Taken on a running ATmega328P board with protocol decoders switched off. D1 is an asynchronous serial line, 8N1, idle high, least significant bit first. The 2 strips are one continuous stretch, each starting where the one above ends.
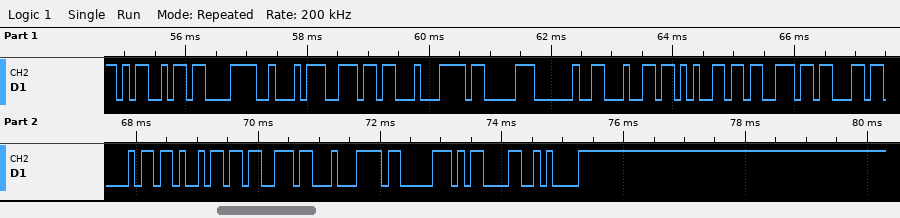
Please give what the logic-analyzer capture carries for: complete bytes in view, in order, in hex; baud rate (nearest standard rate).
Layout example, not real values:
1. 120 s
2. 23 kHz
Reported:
1. 4D C3 A2 6E C4 83 20 64 65 73 63 68 69 73 C4 83 0D 0A
2. 9600 baud
